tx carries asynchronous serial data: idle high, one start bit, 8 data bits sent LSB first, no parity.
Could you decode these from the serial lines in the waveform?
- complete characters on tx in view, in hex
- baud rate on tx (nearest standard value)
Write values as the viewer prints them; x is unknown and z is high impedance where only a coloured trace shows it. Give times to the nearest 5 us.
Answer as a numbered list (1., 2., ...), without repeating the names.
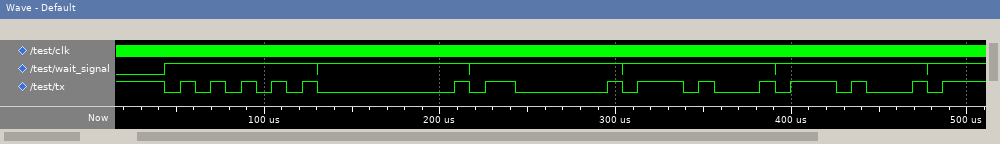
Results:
1. 55, 00, 03, 17, 17
2. 115200 baud
